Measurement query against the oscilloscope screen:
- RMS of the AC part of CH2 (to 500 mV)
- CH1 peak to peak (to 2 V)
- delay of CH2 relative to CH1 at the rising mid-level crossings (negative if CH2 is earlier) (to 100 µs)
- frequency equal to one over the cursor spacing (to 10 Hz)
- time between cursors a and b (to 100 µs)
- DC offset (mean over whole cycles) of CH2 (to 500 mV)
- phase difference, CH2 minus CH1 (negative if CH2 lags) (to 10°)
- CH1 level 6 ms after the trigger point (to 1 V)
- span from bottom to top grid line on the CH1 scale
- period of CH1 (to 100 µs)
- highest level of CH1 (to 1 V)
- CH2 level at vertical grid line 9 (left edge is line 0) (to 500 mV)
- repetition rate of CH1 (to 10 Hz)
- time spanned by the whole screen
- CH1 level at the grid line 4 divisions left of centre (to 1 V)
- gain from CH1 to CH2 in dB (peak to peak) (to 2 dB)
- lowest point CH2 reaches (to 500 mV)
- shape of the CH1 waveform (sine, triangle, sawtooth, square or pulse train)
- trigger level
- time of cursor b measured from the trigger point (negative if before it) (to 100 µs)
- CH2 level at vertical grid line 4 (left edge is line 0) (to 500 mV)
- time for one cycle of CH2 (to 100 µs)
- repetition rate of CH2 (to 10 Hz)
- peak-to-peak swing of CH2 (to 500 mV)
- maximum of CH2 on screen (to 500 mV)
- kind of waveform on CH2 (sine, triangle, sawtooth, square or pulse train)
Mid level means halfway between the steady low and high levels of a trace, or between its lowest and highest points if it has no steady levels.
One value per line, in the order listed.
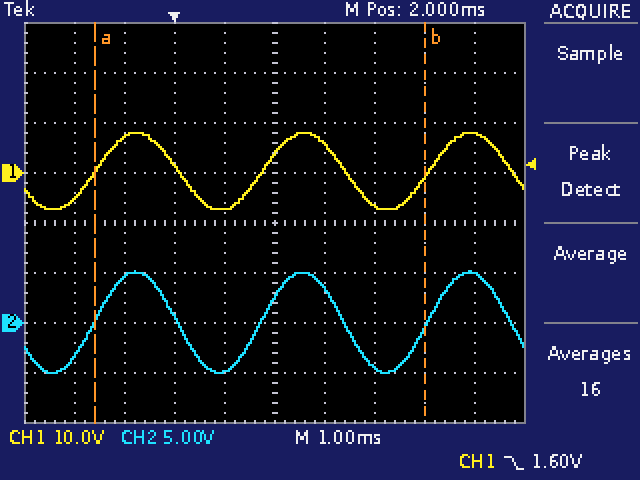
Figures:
3.5 V
16 V
0.0 ms
150 Hz
6.6 ms
0.0 V
0°
8 V
80 V
3.3 ms
8 V
5.0 V
300 Hz
10 ms
-5 V
-4 dB
-5.0 V
sine
1.60 V
+5.0 ms
-5.0 V
3.3 ms
300 Hz
10.0 V
5.0 V
sine
